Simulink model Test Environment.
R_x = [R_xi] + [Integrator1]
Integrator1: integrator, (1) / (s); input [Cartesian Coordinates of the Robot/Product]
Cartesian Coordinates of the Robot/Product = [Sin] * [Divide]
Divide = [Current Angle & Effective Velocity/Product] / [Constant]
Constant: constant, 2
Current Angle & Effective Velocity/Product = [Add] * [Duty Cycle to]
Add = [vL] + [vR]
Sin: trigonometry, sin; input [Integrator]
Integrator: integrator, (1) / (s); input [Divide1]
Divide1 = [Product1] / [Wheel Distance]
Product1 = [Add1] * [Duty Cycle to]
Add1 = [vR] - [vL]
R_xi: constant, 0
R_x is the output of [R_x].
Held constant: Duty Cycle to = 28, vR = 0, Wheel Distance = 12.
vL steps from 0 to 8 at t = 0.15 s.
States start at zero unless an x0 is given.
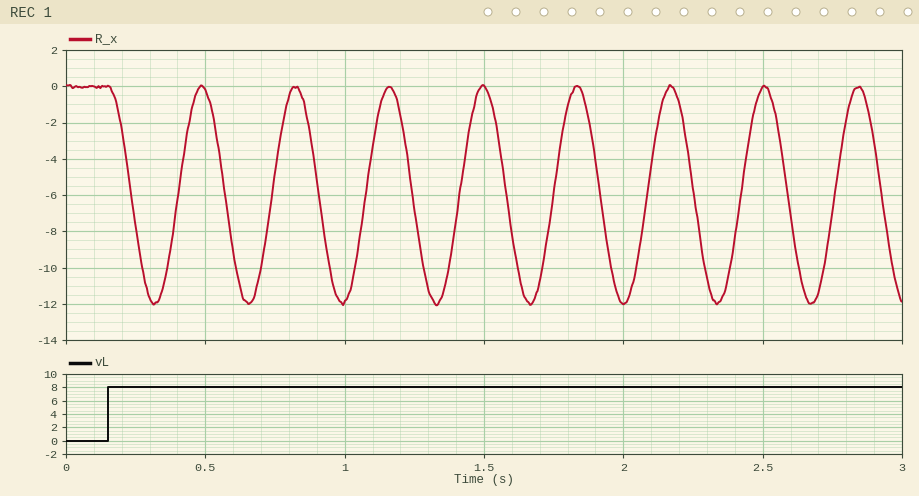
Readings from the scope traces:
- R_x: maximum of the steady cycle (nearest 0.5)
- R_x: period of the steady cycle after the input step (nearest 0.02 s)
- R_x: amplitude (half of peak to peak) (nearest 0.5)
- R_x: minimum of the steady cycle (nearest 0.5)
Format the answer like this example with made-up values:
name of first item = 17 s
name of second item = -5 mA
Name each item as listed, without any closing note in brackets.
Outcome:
R_x: maximum of the steady cycle = 0.0
R_x: period of the steady cycle after the input step = 0.34 s
R_x: amplitude (half of peak to peak) = 6.0
R_x: minimum of the steady cycle = -12.0
